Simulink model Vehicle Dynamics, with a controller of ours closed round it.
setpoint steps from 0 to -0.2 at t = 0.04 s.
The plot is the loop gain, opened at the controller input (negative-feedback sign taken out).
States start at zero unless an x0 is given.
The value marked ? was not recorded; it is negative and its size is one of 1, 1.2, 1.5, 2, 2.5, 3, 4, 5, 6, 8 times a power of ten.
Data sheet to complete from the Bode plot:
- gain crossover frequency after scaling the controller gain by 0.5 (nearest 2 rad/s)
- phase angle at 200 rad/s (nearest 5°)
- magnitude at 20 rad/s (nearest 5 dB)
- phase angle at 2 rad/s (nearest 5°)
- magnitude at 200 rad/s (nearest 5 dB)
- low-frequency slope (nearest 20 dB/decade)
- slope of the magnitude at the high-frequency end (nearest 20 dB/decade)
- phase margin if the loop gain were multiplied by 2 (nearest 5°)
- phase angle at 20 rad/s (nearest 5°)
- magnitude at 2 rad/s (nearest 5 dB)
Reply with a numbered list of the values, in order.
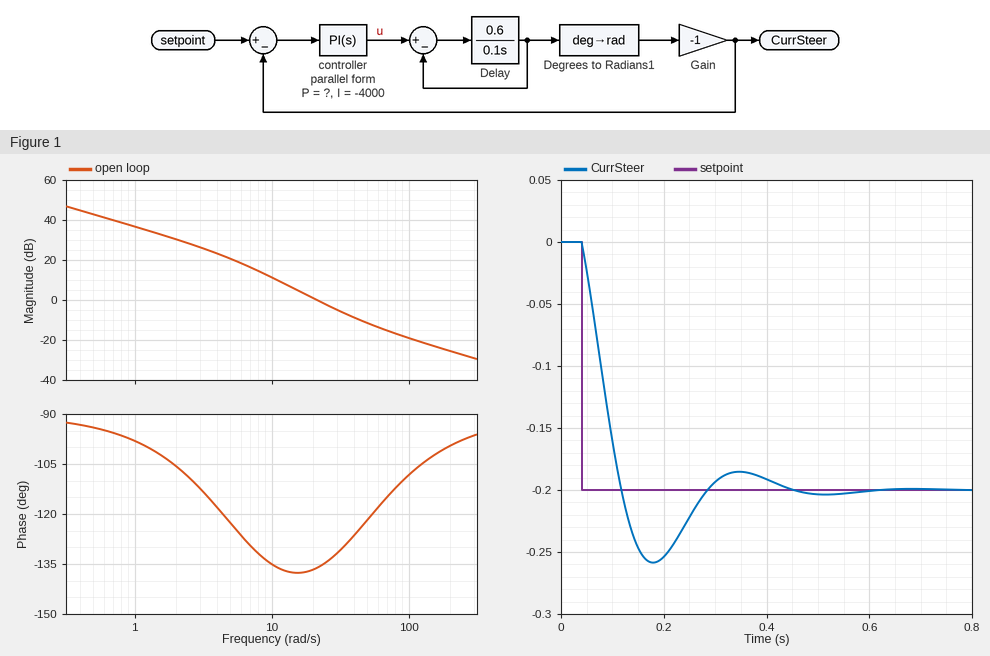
1. 14 rad/s
2. -100°
3. 0 dB
4. -105°
5. -25 dB
6. -20 dB/decade
7. -20 dB/decade
8. 50°
9. -135°
10. 30 dB
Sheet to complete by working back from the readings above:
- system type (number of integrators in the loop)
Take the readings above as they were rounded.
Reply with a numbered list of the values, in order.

1. 1
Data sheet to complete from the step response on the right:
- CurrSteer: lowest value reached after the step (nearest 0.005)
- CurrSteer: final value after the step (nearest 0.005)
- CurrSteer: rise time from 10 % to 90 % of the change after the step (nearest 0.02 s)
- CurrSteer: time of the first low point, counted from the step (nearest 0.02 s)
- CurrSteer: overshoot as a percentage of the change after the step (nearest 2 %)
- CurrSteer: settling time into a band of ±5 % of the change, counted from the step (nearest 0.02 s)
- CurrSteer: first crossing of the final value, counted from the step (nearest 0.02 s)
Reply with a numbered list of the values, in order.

1. -0.260
2. -0.200
3. 0.06 s
4. 0.14 s
5. 30 %
6. 0.36 s
7. 0.08 s
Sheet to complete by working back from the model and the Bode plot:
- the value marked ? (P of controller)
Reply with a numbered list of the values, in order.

1. -100
